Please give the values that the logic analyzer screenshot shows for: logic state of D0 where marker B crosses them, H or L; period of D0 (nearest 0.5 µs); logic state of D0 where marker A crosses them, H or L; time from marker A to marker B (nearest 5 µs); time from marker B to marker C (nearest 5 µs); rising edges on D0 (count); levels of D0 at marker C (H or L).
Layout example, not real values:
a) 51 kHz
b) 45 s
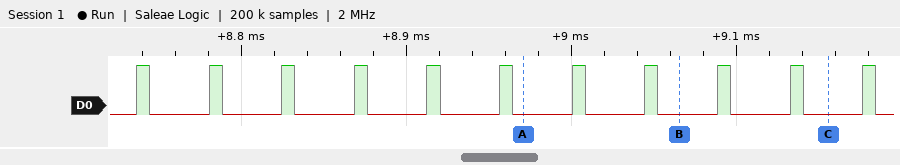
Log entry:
a) D0=L
b) 44 µs
c) D0=L
d) 95 µs
e) 90 µs
f) 11
g) D0=L
